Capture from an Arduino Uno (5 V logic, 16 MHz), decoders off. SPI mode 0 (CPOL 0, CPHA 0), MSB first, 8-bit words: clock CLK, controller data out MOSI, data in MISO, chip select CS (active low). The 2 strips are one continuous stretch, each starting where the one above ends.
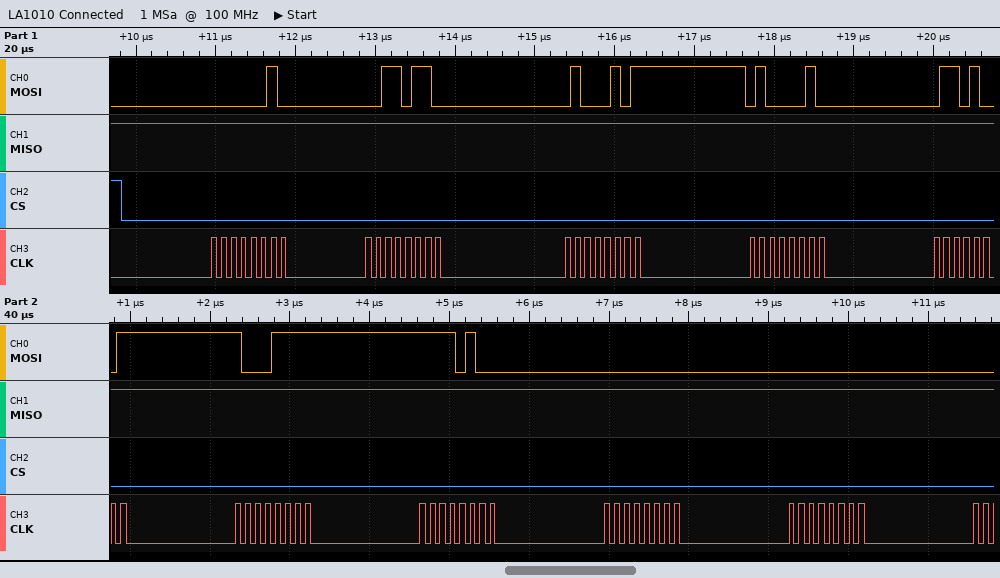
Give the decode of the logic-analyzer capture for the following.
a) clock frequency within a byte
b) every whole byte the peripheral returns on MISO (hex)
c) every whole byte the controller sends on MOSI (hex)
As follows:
8 MHz
0xFF 0xFF 0xFF 0xFF 0xFF 0xFF 0xFF 0xFF 0xFF
0x02 0x36 0x45 0x42 0x69 0x8F 0xF4 0x00 0x00
